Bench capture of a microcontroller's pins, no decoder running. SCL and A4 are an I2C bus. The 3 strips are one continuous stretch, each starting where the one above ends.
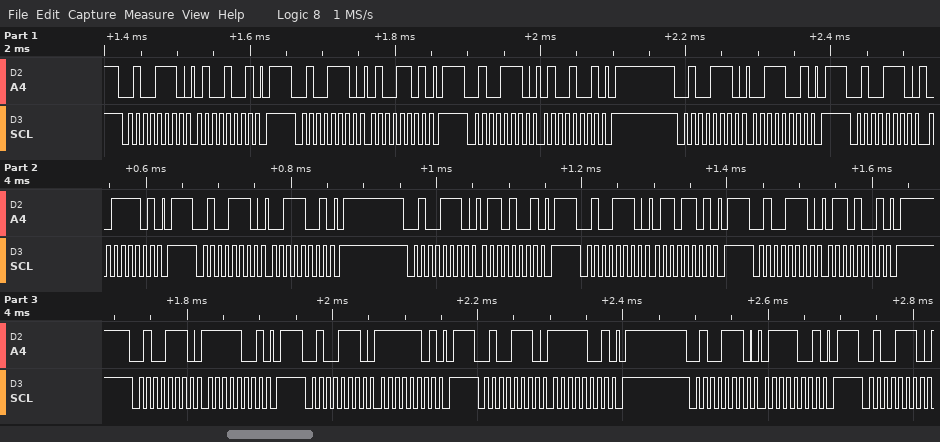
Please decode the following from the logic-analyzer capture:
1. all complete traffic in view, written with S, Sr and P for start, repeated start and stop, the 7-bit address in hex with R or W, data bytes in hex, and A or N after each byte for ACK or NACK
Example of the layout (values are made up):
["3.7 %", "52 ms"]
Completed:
["S 27W A 49 A P S 27W A 4D A P S 27W A 49 A P S 27W A 39 A P S 27W A 3D A P S 27W A 39 A P S 27W A 69 A P S 27W A 6D A P S 27W A 69 A P S 27W A F9 A P S 27W A FD A P S 27W A F9 A P S 27W A 79 A P S 27W A"]
